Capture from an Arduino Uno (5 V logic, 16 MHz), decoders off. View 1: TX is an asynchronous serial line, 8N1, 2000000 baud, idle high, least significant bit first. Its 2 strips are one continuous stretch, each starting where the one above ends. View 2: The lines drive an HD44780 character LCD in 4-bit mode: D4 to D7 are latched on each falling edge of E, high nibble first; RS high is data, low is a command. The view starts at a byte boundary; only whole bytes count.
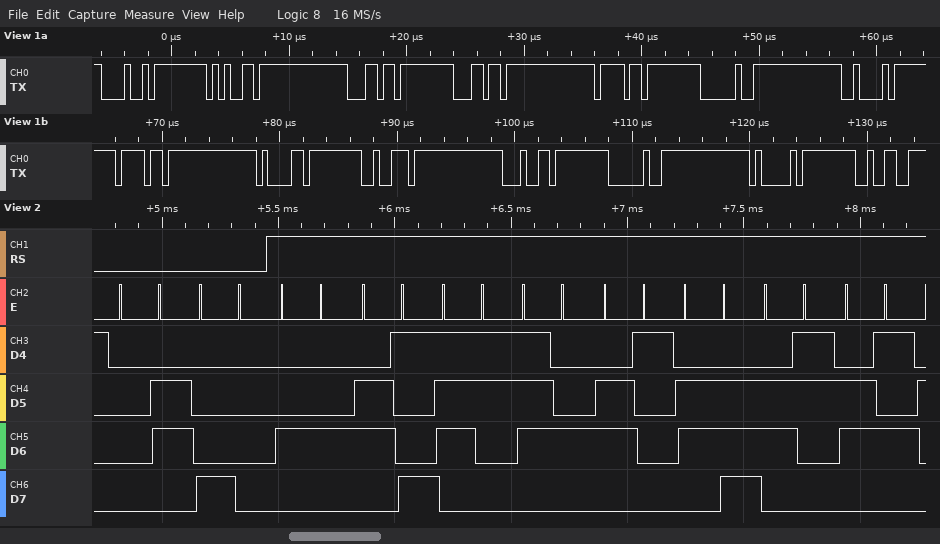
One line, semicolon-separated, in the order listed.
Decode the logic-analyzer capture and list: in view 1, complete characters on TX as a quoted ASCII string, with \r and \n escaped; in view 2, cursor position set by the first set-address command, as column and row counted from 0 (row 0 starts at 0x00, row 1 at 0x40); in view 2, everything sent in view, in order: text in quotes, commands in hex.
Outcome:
"Hello Board A2"; column 0, row 0; 0x06 0x80 "Distance"
